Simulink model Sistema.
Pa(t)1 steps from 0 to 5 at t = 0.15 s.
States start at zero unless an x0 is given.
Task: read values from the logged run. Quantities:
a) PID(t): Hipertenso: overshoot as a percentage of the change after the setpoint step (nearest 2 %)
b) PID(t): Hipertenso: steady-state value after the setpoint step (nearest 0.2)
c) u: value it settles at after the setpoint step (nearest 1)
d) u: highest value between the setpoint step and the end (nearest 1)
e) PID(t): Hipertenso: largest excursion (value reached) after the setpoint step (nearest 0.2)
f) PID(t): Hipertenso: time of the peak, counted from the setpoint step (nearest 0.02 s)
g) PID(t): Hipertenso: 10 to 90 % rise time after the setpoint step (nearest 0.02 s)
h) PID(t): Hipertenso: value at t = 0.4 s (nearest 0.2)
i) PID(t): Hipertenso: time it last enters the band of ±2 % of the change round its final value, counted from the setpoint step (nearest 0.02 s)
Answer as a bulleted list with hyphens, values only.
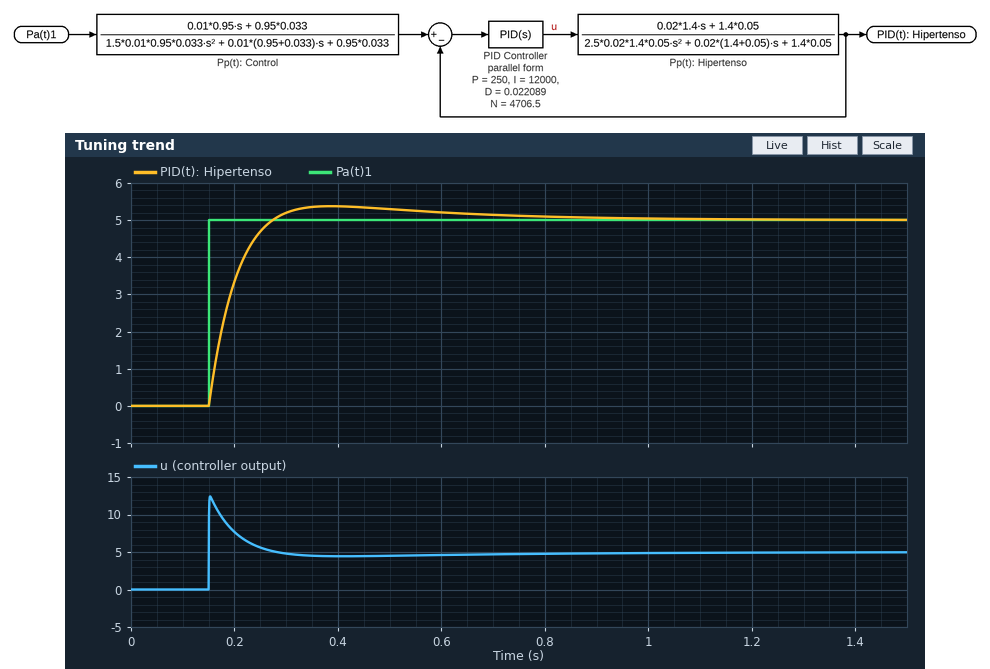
- 8 %
- 5.0
- 5
- 12
- 5.4
- 0.24 s
- 0.08 s
- 5.4
- 0.64 s
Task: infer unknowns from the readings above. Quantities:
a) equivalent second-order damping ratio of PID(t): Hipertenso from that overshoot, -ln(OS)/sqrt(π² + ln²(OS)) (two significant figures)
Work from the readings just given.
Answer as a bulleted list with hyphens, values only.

- 0.63
